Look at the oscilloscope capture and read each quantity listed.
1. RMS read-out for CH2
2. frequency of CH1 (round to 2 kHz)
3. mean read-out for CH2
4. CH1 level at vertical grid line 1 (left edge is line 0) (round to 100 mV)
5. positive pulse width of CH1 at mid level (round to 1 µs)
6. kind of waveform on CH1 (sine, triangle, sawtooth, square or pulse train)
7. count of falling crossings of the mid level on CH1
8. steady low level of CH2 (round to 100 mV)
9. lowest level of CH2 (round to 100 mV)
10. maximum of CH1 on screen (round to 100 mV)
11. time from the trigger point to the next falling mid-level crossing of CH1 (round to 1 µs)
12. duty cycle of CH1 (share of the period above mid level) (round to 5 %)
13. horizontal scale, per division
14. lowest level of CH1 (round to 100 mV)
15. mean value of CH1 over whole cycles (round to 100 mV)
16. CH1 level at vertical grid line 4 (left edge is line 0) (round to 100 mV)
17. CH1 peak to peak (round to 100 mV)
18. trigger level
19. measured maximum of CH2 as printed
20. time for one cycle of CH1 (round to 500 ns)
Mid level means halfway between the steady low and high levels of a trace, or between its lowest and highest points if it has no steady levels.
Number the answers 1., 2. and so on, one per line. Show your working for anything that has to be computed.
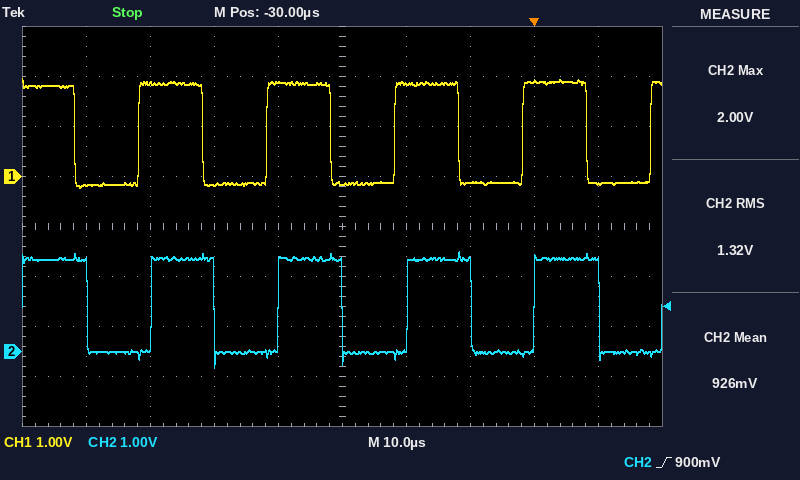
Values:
1. 1.32 V
2. 1 / 20.0 µs ≈ 50 kHz
3. 926 mV
4. -200 mV
5. 10 µs
6. square
7. 5
8. 0.0 V
9. -300 mV
10. 2.0 V
11. 8 µs
12. 10 µs / 20.0 µs ≈ 50 %
13. 10 µs
14. -200 mV
15. -200 mV + 0.5 × (2.0 V − (-200 mV)) ≈ 900 mV
16. 1.9 V
17. 2.0 V − (-200 mV) = 2.2 V
18. 900 mV
19. 2.00 V
20. 20.0 µs
